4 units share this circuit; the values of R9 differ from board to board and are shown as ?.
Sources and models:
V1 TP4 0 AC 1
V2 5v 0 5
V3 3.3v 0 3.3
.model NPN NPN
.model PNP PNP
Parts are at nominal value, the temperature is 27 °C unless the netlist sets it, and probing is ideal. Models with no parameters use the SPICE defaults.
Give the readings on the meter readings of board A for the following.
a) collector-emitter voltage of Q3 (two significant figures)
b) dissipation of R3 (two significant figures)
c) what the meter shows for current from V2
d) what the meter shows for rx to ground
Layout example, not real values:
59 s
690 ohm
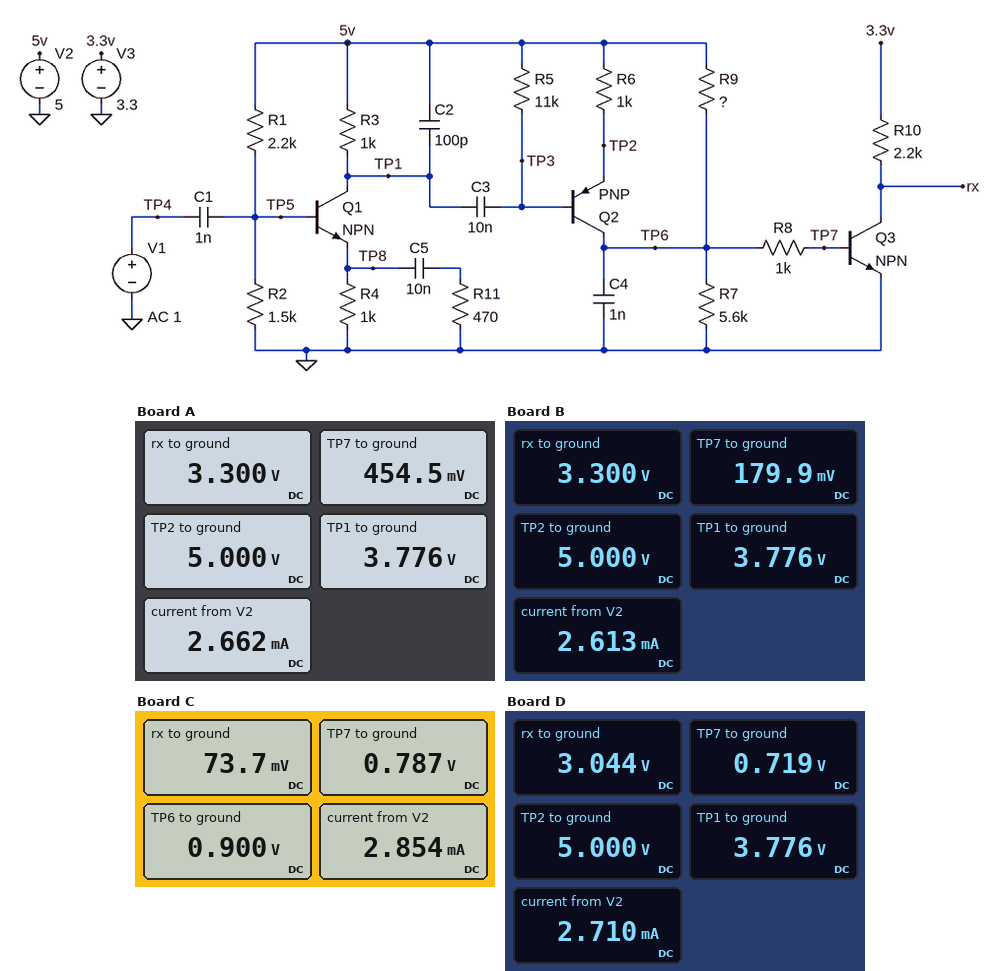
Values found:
3.3 V
1.5 mW
2.662 mA
3.300 V
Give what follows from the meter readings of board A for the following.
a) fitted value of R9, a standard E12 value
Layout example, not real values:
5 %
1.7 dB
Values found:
56 kΩ
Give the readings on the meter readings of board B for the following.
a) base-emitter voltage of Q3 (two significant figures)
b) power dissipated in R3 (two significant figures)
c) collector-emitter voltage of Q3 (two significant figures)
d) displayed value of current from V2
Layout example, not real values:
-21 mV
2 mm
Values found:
180 mV
1.5 mW
3.3 V
2.613 mA
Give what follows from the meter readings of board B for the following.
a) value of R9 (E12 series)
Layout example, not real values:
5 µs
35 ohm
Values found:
150 kΩ
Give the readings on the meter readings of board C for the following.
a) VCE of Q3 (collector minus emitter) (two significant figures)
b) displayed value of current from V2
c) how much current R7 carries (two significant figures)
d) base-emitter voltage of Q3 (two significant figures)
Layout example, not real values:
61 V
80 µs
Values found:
74 mV
2.854 mA
160 µA
790 mV
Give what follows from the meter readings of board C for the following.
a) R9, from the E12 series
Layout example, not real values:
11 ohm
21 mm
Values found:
15 kΩ
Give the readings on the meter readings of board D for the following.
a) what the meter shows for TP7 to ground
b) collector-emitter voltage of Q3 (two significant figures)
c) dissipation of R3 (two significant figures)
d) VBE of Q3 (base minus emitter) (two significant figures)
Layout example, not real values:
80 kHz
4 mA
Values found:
0.719 V
3.0 V
1.5 mW
720 mV
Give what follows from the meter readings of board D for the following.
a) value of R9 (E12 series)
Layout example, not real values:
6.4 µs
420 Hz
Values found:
33 kΩ
